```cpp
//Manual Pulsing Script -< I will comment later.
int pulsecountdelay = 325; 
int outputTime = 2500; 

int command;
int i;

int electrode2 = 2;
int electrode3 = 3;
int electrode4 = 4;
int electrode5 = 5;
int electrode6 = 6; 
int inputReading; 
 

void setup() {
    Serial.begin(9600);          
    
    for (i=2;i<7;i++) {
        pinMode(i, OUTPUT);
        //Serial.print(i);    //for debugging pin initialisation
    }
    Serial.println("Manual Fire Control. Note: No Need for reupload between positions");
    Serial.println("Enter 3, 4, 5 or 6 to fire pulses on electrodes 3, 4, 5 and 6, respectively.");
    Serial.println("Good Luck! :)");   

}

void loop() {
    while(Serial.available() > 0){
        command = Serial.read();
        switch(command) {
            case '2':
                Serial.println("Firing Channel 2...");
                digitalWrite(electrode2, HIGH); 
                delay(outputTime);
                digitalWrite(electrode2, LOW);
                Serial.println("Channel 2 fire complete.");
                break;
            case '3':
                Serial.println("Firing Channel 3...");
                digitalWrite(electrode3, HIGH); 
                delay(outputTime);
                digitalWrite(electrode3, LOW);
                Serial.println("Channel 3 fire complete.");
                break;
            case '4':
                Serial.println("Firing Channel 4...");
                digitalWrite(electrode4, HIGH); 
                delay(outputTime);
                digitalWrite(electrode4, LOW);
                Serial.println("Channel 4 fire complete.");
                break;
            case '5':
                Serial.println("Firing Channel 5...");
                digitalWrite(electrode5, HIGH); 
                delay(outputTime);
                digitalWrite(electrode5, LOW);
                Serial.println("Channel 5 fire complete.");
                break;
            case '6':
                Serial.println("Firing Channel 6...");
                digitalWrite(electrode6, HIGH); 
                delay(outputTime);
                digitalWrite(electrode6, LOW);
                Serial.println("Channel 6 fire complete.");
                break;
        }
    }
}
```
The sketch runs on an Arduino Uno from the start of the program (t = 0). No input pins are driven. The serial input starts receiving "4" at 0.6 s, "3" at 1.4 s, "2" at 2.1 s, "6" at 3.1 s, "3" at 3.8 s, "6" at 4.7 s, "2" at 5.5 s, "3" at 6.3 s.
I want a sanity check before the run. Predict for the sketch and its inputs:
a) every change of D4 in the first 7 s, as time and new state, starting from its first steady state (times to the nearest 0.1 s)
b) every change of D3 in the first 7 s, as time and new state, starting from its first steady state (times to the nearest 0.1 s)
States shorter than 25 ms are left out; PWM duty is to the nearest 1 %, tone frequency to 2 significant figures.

0 s low; 0.6 s high; 3.1 s low
0 s low; 3.1 s high; 5.6 s low
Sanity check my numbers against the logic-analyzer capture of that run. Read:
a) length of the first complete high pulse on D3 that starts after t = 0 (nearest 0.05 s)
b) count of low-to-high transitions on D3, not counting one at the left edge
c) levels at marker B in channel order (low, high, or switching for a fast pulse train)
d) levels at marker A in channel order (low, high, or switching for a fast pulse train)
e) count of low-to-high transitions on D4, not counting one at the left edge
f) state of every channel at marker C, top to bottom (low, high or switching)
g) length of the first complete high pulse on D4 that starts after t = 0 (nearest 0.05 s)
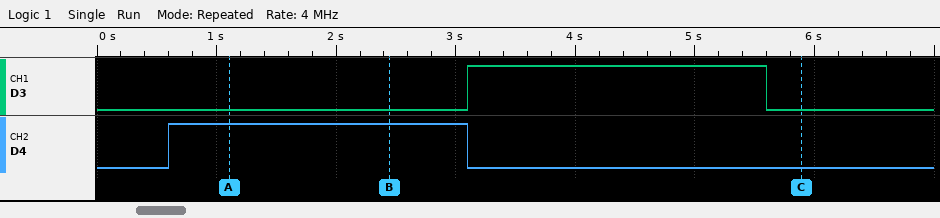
2.50 s
1
D3 low, D4 high
D3 low, D4 high
1
D3 low, D4 low
2.50 s
